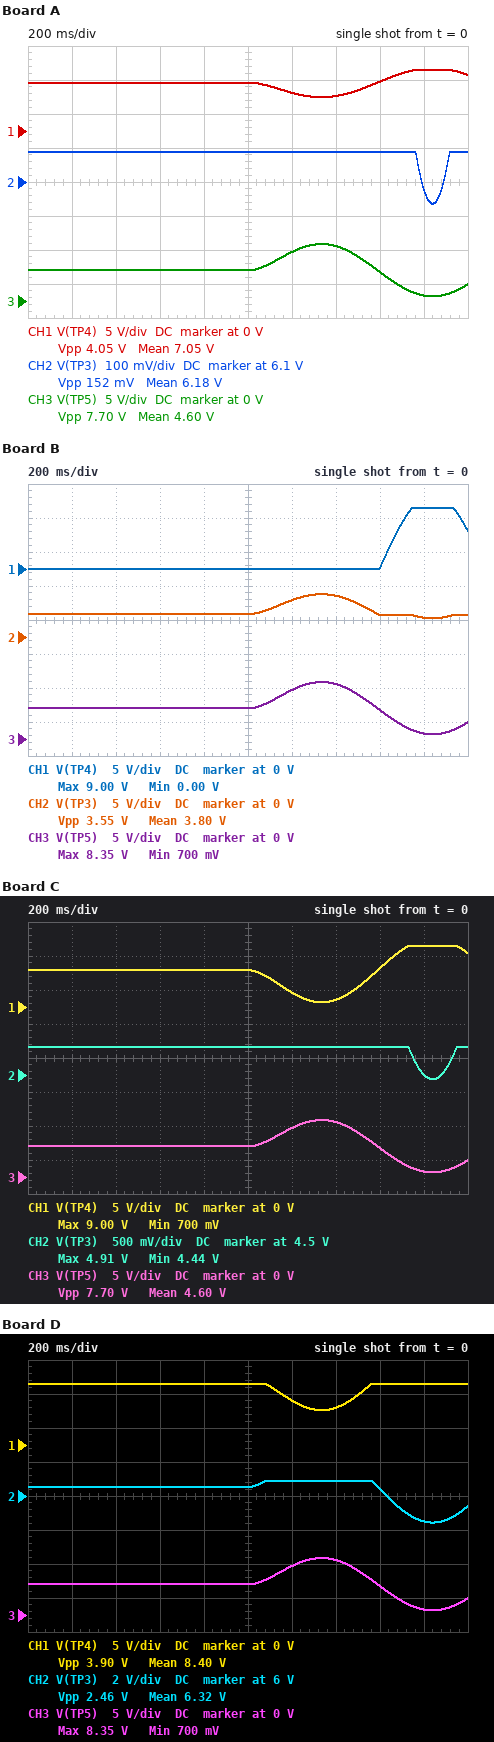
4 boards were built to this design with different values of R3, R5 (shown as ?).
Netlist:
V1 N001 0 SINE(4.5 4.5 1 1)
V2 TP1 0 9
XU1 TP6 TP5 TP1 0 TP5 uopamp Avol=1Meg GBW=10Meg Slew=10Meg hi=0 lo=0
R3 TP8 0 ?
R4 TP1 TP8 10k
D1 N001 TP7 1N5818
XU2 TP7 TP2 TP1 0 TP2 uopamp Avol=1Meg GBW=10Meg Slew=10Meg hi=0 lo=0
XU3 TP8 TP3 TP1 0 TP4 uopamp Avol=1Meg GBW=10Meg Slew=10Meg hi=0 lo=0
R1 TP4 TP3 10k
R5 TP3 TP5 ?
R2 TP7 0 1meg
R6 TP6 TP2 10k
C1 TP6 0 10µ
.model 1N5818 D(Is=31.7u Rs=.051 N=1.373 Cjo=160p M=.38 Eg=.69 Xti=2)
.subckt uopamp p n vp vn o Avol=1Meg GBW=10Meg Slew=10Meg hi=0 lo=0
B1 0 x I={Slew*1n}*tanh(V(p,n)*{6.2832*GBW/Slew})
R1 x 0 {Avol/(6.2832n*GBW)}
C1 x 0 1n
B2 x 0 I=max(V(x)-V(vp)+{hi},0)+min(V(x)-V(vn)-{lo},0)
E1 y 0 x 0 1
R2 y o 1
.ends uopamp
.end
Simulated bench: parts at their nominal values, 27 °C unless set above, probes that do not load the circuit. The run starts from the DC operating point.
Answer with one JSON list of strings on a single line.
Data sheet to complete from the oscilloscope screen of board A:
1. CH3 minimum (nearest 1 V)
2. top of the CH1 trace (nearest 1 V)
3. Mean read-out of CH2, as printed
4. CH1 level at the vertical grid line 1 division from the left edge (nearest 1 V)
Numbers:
["1 V", "9 V", "6.18 V", "7 V"]
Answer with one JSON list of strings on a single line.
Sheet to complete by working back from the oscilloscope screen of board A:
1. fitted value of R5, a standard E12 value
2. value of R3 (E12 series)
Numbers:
["18 kΩ", "22 kΩ"]
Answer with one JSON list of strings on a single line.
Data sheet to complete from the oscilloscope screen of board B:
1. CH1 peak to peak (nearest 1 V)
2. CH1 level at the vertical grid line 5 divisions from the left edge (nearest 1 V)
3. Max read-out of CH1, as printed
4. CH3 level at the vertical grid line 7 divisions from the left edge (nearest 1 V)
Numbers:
["9 V", "0 V", "9.00 V", "8 V"]
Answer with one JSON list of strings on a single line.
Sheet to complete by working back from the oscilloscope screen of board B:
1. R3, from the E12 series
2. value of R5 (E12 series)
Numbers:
["5.6 kΩ", "3.3 kΩ"]
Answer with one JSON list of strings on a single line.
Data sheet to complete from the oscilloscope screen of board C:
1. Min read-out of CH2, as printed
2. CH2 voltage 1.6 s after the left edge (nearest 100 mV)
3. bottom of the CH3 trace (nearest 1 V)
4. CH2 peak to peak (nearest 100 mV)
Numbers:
["4.44 V", "4.9 V", "1 V", "500 mV"]
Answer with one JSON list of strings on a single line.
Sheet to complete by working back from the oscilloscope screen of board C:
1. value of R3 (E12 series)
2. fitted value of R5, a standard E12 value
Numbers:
["12 kΩ", "8.2 kΩ"]
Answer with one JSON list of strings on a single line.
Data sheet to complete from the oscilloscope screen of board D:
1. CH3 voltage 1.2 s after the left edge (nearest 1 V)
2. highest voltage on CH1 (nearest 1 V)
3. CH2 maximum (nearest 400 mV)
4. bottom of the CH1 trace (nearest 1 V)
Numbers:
["7 V", "9 V", "6.8 V", "5 V"]
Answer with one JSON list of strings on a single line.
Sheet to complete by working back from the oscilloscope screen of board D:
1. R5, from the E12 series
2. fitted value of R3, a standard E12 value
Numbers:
["8.2 kΩ", "33 kΩ"]
